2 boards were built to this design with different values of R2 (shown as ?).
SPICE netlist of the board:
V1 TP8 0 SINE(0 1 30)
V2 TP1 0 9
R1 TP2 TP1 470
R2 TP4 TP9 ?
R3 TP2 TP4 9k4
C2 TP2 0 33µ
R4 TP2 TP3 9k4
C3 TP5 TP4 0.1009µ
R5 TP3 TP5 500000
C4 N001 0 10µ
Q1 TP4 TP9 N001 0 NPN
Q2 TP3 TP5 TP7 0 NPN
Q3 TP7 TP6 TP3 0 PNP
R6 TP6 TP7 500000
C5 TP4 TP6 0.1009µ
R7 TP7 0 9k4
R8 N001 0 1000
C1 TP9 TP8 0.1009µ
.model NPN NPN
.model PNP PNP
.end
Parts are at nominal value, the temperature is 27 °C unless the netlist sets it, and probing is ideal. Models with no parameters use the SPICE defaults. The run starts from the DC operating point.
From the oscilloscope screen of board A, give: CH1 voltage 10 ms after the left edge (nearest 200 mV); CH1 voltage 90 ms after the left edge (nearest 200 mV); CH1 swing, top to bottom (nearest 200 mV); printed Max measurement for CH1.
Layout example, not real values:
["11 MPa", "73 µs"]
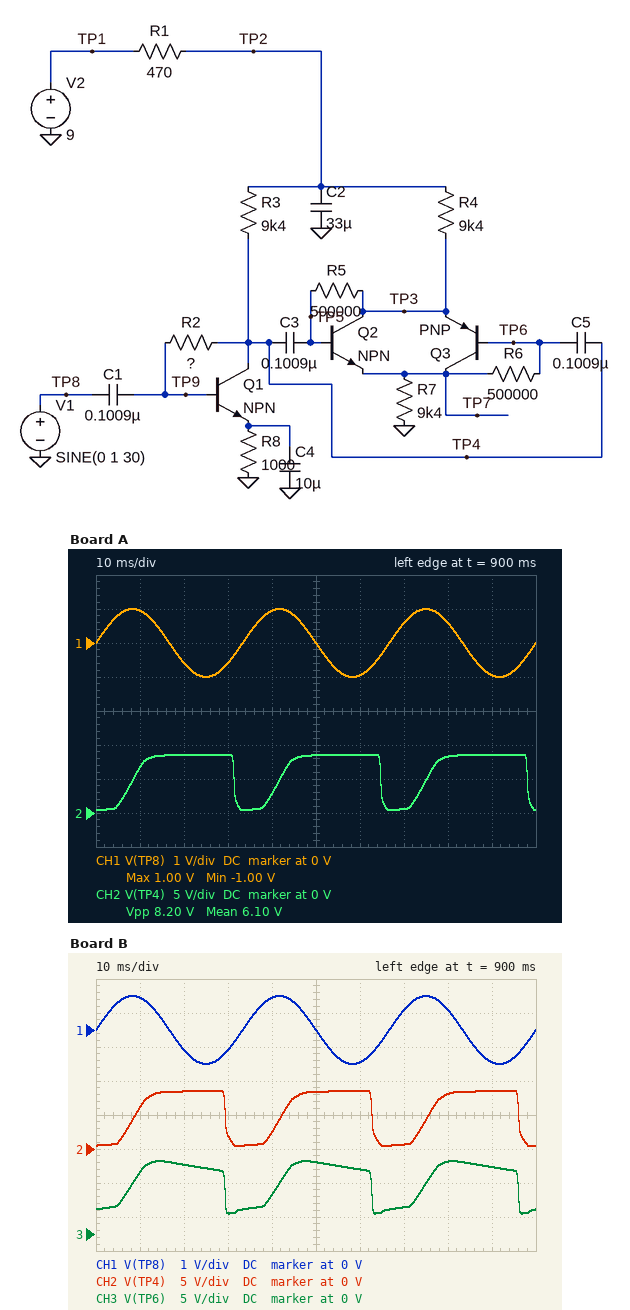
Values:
["1.0 V", "-1.0 V", "2.0 V", "1.00 V"]
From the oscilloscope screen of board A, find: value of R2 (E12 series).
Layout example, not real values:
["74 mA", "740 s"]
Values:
["1.8 MΩ"]
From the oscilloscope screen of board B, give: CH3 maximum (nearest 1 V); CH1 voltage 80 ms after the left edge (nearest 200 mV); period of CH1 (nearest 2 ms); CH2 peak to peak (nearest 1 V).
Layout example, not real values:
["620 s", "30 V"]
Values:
["11 V", "600 mV", "34 ms", "8 V"]
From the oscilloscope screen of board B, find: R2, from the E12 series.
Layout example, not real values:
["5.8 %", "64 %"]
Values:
["1.2 MΩ"]
